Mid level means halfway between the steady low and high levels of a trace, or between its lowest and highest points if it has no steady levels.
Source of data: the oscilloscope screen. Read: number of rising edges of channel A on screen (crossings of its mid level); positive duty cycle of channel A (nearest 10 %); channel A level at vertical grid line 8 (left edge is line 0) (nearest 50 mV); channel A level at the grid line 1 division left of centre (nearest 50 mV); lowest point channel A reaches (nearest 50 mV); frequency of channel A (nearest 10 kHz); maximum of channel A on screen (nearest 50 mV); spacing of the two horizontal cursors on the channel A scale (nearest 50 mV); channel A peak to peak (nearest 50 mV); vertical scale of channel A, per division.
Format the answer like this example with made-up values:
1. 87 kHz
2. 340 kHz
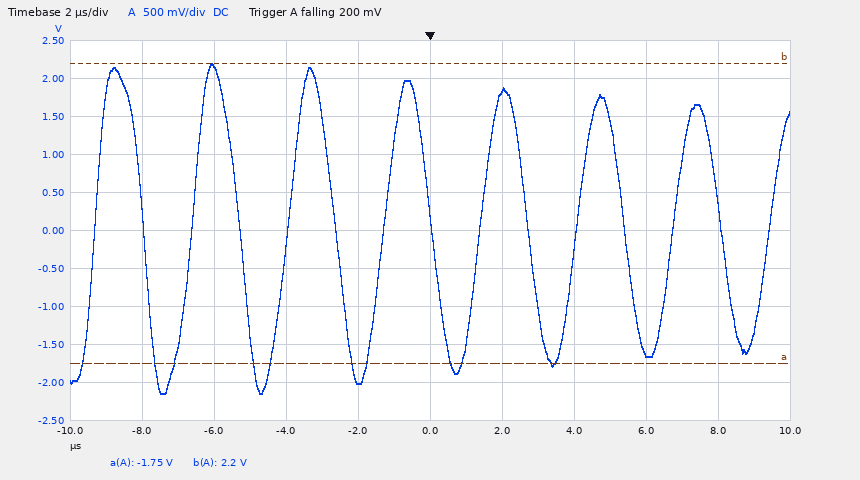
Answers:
1. 8
2. 50 %
3. -1.60 V
4. -2.00 V
5. -2.15 V
6. 370 kHz
7. 2.20 V
8. 3.95 V
9. 4.35 V
10. 500 mV
